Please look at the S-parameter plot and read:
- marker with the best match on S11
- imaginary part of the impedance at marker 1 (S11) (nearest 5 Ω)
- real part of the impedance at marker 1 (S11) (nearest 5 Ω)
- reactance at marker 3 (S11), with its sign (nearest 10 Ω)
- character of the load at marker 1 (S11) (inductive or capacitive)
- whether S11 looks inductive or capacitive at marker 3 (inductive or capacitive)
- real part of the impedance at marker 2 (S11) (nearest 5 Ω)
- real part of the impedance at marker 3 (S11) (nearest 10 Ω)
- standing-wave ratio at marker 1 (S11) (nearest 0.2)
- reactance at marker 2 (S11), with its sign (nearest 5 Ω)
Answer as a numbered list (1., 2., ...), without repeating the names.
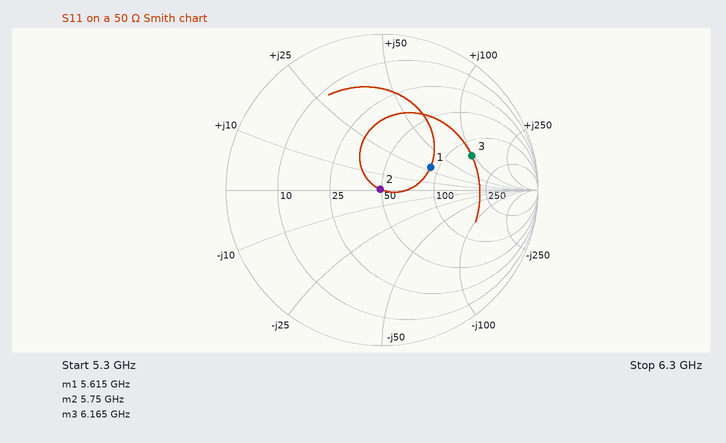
1. marker 2
2. +30 Ω
3. 90 Ω
4. +100 Ω
5. inductive
6. inductive
7. 50 Ω
8. 140 Ω
9. 2.0
10. 0 Ω
